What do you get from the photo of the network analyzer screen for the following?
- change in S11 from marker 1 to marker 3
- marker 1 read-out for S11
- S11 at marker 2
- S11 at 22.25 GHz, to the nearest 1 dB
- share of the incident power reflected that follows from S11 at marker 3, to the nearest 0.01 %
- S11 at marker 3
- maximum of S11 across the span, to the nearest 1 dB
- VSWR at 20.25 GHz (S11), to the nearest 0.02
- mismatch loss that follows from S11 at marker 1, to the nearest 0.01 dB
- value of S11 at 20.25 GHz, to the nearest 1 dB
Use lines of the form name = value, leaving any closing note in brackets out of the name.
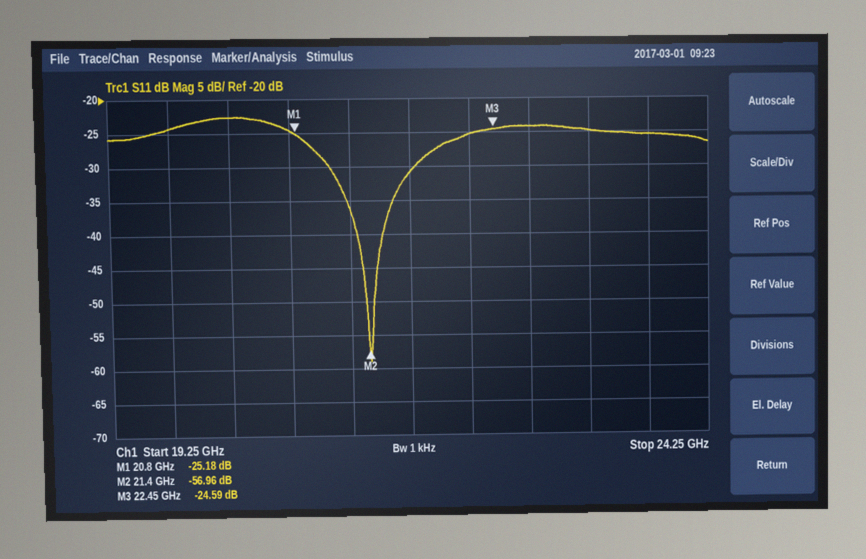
change in S11 from marker 1 to marker 3 = 0.59 dB
marker 1 read-out for S11 = -25.18 dB
S11 at marker 2 = -56.96 dB
S11 at 22.25 GHz, to the nearest 1 dB = -25 dB
share of the incident power reflected that follows from S11 at marker 3, to the nearest 0.01 % = 0.35 %
S11 at marker 3 = -24.59 dB
maximum of S11 across the span, to the nearest 1 dB = -23 dB
VSWR at 20.25 GHz (S11), to the nearest 0.02 = 1.16
mismatch loss that follows from S11 at marker 1, to the nearest 0.01 dB = 0.01 dB
value of S11 at 20.25 GHz, to the nearest 1 dB = -23 dB
